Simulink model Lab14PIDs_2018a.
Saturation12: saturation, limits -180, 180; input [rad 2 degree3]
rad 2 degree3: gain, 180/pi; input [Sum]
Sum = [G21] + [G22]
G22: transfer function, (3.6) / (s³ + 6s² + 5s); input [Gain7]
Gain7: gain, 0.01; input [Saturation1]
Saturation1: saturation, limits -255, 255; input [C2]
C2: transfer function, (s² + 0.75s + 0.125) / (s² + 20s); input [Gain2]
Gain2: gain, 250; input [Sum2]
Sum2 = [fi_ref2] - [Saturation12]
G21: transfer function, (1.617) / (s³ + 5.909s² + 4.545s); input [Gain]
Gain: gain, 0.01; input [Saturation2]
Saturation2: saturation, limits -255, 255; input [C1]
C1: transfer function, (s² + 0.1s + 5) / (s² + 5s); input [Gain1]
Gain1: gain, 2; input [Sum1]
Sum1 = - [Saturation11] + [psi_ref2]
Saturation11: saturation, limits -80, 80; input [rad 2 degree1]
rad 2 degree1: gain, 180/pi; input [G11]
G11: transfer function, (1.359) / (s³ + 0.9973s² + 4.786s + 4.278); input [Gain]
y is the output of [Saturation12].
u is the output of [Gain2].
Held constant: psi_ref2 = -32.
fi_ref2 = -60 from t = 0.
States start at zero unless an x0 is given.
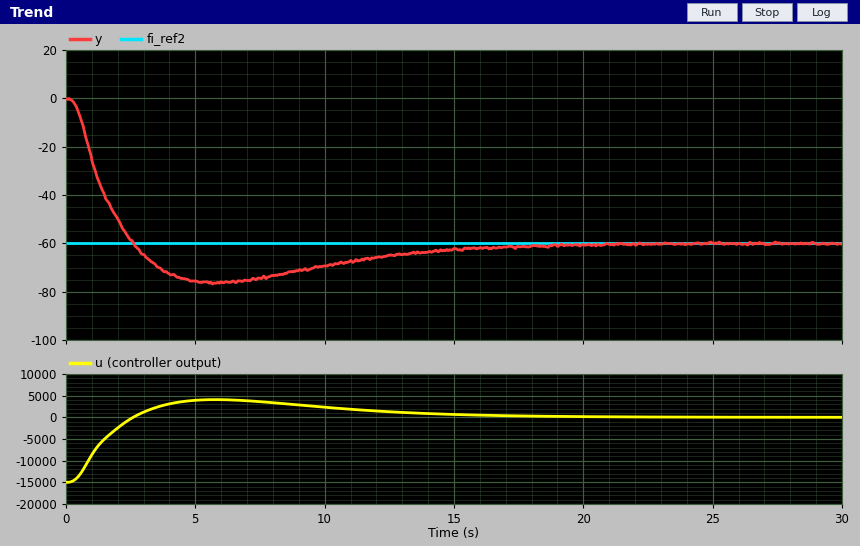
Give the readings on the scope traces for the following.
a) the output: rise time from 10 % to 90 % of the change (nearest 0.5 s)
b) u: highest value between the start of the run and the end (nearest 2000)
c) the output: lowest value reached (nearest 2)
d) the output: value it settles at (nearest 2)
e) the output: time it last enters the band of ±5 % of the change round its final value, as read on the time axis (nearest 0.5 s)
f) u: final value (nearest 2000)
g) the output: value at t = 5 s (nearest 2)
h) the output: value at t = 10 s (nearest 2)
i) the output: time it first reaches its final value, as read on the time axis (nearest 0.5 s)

1.5 s
4000
-76
-60
14.5 s
0
-76
-70
2.5 s
